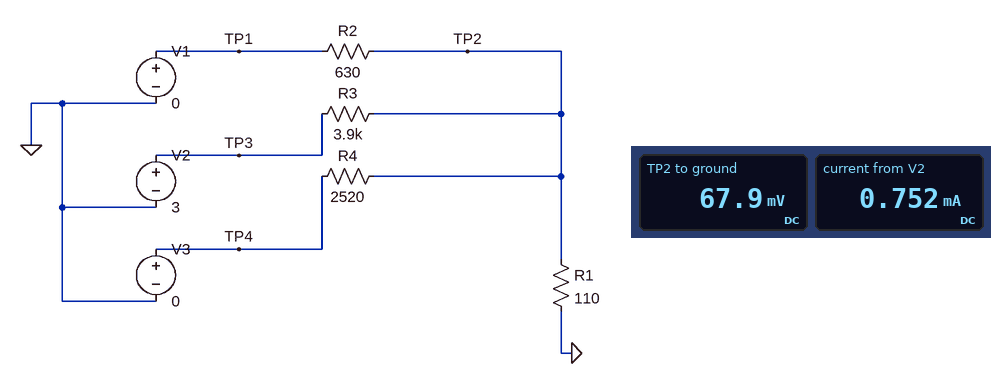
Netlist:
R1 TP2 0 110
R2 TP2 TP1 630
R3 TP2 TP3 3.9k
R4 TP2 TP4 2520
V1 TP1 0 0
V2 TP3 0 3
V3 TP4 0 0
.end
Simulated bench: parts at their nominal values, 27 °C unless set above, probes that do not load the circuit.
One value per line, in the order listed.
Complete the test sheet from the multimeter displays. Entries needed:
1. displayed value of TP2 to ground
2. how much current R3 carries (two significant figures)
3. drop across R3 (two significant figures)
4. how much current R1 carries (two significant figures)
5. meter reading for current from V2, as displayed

67.9 mV
750 µA
2.9 V
620 µA
0.752 mA
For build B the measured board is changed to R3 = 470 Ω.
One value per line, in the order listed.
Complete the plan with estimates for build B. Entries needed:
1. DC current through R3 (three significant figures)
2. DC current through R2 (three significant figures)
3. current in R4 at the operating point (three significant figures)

5.35 mA
767 µA
192 µA
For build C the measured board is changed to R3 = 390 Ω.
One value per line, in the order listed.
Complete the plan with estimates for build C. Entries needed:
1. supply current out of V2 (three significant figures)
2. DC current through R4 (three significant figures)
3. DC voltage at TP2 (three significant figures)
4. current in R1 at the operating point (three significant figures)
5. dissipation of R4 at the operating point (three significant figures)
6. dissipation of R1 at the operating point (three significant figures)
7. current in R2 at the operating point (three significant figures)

6.25 mA
224 µA
564 mV
5.13 mA
126 µW
2.89 mW
895 µA
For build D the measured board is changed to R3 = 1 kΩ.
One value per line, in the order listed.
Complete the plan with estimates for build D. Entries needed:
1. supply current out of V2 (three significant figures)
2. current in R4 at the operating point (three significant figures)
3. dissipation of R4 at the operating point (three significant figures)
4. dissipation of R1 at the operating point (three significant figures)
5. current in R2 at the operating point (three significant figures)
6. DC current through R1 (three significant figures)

2.75 mA
98.6 µA
24.5 µW
561 µW
394 µA
2.26 mA
